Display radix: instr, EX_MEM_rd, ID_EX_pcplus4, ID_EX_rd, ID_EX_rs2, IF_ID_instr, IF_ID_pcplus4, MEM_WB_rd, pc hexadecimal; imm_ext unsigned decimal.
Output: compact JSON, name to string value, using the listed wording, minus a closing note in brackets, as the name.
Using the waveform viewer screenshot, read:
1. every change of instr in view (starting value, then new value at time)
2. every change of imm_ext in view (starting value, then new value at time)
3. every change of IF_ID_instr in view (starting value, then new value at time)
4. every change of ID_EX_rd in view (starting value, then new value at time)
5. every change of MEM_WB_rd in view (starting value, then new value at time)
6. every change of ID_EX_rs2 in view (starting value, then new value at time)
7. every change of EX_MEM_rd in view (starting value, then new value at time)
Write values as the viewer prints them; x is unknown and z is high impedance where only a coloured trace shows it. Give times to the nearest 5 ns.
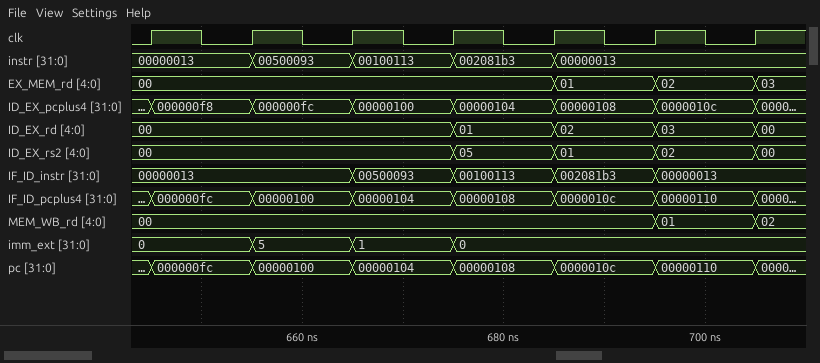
{"every change of instr in view": "00000013, 00500093 at 655 ns, 00100113 at 665 ns, 002081b3 at 675 ns, 00000013 at 685 ns", "every change of imm_ext in view": "0, 5 at 655 ns, 1 at 665 ns, 0 at 675 ns", "every change of IF_ID_instr in view": "00000013, 00500093 at 665 ns, 00100113 at 675 ns, 002081b3 at 685 ns, 00000013 at 695 ns", "every change of ID_EX_rd in view": "00, 01 at 675 ns, 02 at 685 ns, 03 at 695 ns, 00 at 705 ns", "every change of MEM_WB_rd in view": "00, 01 at 695 ns, 02 at 705 ns", "every change of ID_EX_rs2 in view": "00, 05 at 675 ns, 01 at 685 ns, 02 at 695 ns, 00 at 705 ns", "every change of EX_MEM_rd in view": "00, 01 at 685 ns, 02 at 695 ns, 03 at 705 ns"}
